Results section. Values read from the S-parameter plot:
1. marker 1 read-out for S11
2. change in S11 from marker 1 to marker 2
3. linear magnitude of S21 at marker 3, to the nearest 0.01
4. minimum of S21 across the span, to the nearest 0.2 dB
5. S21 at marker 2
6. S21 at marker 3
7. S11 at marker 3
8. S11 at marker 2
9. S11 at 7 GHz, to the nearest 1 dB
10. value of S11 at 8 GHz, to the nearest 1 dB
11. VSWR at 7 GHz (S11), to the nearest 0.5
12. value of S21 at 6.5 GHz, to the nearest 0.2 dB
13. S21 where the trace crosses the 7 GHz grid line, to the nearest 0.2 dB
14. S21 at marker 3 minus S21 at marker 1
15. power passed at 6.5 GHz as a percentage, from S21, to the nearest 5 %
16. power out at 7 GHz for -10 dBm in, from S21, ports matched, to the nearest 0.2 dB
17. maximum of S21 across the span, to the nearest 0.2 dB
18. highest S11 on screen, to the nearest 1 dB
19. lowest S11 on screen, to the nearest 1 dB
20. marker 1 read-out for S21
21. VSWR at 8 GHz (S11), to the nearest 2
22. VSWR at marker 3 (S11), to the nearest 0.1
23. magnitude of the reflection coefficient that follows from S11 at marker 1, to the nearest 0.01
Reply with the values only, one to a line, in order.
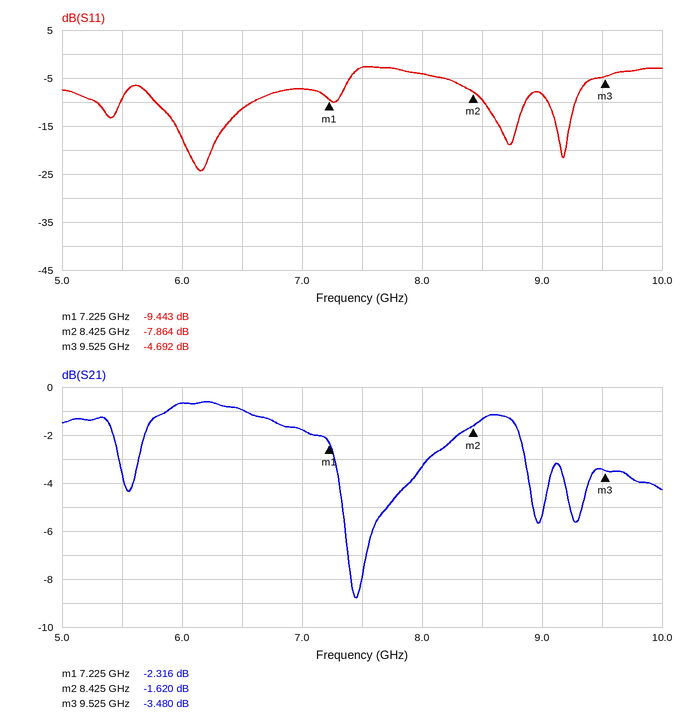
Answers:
-9.443 dB
1.579 dB
0.67
-8.8 dB
-1.620 dB
-3.480 dB
-4.692 dB
-7.864 dB
-7 dB
-4 dB
2.5
-1.0 dB
-1.8 dB
-1.164 dB
80 %
-11.8 dBm
-0.6 dB
-3 dB
-24 dB
-2.316 dB
4
3.8
0.34
